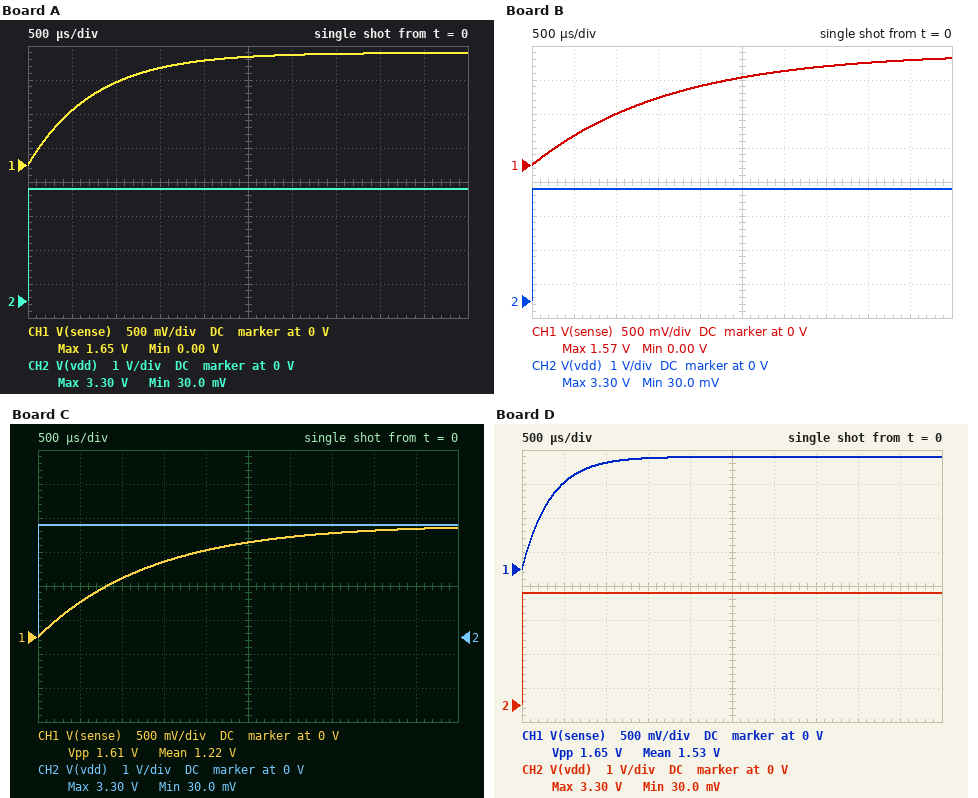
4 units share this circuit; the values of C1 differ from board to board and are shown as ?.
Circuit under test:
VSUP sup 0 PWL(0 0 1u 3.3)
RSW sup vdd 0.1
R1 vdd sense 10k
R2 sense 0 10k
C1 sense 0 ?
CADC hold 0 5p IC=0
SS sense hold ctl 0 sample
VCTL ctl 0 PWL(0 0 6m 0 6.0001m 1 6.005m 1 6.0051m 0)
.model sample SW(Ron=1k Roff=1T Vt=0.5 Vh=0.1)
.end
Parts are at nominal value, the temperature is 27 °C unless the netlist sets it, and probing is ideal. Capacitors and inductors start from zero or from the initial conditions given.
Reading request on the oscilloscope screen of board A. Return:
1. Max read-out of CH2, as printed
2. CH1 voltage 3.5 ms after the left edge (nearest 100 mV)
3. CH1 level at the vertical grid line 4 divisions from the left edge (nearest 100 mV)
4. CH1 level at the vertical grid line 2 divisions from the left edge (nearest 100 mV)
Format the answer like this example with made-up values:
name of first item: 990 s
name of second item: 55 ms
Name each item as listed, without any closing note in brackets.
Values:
Max read-out of CH2, as printed: 3.30 V
CH1 voltage 3.5 ms after the left edge: 1.6 V
CH1 level at the vertical grid line 4 divisions from the left edge: 1.5 V
CH1 level at the vertical grid line 2 divisions from the left edge: 1.2 V
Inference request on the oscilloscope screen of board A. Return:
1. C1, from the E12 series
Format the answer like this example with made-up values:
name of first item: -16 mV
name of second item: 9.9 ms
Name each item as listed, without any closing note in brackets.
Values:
C1, from the E12 series: 150 nF
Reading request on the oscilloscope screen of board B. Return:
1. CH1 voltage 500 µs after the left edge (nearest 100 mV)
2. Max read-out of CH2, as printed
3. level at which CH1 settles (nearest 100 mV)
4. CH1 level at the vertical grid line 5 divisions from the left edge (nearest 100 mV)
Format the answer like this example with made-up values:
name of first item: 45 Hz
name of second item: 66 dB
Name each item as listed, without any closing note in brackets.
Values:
CH1 voltage 500 µs after the left edge: 400 mV
Max read-out of CH2, as printed: 3.30 V
level at which CH1 settles: 1.6 V
CH1 level at the vertical grid line 5 divisions from the left edge: 1.3 V
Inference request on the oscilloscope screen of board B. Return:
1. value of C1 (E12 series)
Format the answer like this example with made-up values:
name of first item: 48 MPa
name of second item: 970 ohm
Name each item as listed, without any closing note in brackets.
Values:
value of C1: 330 nF
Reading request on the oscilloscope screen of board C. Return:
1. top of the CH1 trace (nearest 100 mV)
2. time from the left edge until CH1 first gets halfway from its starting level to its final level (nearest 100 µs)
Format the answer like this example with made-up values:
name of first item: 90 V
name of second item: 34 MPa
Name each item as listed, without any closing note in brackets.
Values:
top of the CH1 trace: 1.6 V
time from the left edge until CH1 first gets halfway from its starting level to its final level: 900 µs
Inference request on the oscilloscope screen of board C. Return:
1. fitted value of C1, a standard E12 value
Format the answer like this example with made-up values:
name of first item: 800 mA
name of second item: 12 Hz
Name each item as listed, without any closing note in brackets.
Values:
fitted value of C1, a standard E12 value: 270 nF
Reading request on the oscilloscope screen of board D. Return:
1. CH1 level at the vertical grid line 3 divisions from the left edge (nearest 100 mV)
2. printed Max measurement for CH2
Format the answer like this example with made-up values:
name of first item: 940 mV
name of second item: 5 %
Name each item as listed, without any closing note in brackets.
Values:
CH1 level at the vertical grid line 3 divisions from the left edge: 1.6 V
printed Max measurement for CH2: 3.30 V
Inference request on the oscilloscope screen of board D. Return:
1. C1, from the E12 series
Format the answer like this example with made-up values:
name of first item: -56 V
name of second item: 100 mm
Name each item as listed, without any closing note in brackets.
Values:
C1, from the E12 series: 68 nF
